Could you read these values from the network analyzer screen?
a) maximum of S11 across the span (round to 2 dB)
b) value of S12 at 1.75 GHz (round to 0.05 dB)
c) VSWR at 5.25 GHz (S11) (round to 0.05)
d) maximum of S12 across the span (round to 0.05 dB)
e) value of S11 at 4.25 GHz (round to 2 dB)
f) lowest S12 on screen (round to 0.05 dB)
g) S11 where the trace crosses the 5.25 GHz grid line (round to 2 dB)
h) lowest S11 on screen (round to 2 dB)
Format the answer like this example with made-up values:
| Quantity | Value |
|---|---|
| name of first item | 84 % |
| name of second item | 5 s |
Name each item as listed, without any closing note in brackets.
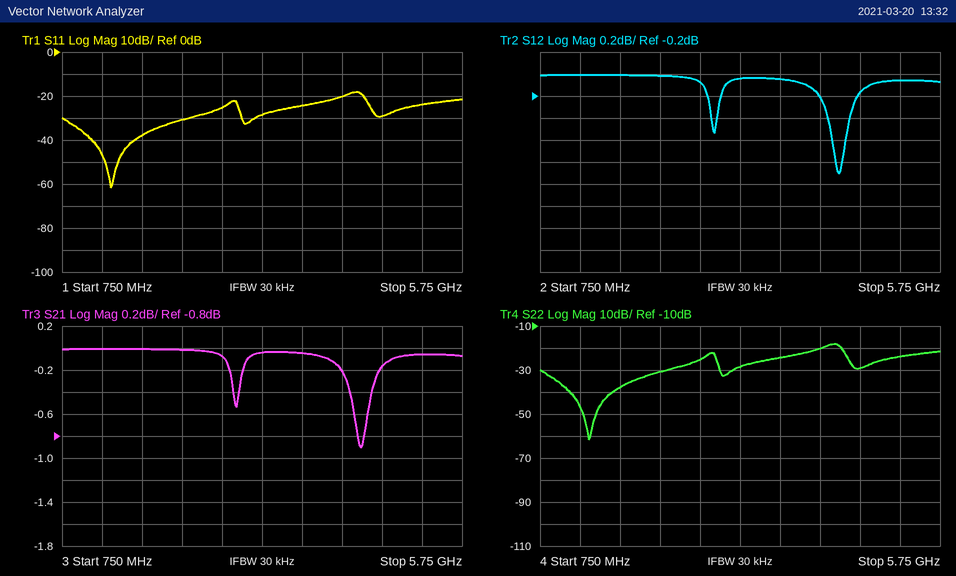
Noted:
| Quantity | Value |
|---|---|
| maximum of S11 across the span | -18 dB |
| value of S12 at 1.75 GHz | 0.00 dB |
| VSWR at 5.25 GHz (S11) | 1.15 |
| maximum of S12 across the span | 0.00 dB |
| value of S11 at 4.25 GHz | -20 dB |
| lowest S12 on screen | -0.90 dB |
| S11 where the trace crosses the 5.25 GHz grid line | -24 dB |
| lowest S11 on screen | -62 dB |
